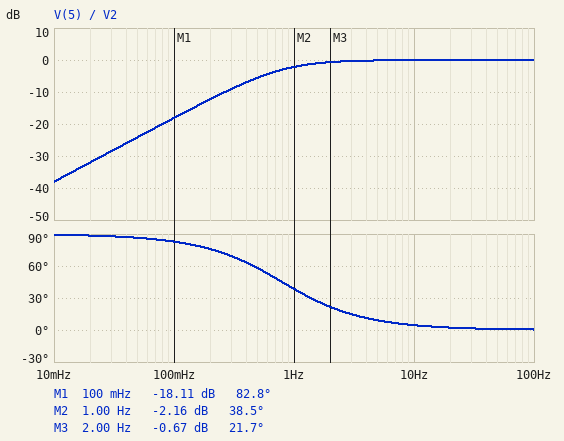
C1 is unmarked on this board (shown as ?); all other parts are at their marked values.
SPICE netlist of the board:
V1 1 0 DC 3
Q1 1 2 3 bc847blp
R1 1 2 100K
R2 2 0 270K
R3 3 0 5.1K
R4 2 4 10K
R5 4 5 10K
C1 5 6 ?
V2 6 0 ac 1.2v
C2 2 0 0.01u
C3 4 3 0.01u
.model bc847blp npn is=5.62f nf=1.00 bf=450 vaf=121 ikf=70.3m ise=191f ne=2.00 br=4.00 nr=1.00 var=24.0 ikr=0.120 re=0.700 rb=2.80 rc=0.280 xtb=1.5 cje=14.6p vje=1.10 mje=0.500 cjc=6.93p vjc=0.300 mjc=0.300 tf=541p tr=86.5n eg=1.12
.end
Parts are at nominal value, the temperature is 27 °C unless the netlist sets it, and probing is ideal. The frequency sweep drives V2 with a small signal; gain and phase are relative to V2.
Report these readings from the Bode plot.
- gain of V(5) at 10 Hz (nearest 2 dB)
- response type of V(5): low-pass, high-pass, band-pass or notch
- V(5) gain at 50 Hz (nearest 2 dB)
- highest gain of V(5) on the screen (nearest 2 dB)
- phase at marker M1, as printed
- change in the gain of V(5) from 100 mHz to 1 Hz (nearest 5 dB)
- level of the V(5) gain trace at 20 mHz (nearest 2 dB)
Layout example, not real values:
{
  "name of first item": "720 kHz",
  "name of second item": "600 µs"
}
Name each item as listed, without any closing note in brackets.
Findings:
{
  "gain of V(5) at 10 Hz": "0 dB",
  "response type of V(5): low-pass, high-pass, band-pass or notch": "high-pass",
  "V(5) gain at 50 Hz": "0 dB",
  "highest gain of V(5) on the screen": "0 dB",
  "phase at marker M1, as printed": "82.8 deg",
  "change in the gain of V(5) from 100 mHz to 1 Hz": "15 dB",
  "level of the V(5) gain trace at 20 mHz": "-32 dB"
}
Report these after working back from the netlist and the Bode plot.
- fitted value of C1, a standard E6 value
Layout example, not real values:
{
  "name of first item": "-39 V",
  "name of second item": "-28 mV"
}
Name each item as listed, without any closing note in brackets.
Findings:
{
  "fitted value of C1, a standard E6 value": "2.2 µF"
}
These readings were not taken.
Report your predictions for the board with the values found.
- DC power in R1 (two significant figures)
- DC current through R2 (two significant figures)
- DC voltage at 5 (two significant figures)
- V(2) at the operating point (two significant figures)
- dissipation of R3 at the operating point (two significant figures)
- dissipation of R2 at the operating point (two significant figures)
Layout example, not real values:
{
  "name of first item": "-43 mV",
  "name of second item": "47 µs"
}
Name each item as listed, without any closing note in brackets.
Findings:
{
  "DC power in R1": "7.4 µW",
  "DC current through R2": "7.9 µA",
  "DC voltage at 5": "2.1 V",
  "V(2) at the operating point": "2.1 V",
  "dissipation of R3 at the operating point": "440 µW",
  "dissipation of R2 at the operating point": "17 µW"
}
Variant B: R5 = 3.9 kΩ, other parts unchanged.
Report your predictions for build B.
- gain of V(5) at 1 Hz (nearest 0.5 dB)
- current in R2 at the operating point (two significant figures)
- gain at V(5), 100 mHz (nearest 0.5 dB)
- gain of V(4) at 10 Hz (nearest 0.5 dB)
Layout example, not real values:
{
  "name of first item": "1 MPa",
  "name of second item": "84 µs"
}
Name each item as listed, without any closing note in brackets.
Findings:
{
  "gain of V(5) at 1 Hz": "-2.5 dB",
  "current in R2 at the operating point": "7.9 µA",
  "gain at V(5), 100 mHz": "-18.5 dB",
  "gain of V(4) at 10 Hz": "-0.5 dB"
}
